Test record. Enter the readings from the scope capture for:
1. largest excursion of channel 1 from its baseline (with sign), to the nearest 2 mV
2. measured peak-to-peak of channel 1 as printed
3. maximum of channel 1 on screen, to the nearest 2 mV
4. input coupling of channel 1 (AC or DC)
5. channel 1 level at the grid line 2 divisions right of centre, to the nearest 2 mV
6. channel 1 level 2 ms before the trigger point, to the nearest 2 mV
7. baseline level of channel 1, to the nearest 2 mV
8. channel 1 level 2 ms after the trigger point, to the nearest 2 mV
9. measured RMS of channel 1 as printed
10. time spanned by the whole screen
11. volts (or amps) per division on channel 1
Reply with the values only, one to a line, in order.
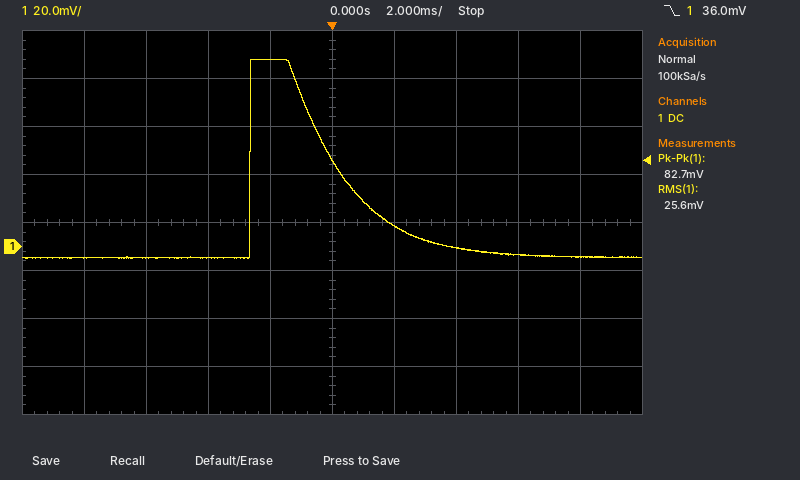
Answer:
+82 mV
82.7 mV
78 mV
DC
0 mV
78 mV
-4 mV
8 mV
25.6 mV
20 ms
20 mV
